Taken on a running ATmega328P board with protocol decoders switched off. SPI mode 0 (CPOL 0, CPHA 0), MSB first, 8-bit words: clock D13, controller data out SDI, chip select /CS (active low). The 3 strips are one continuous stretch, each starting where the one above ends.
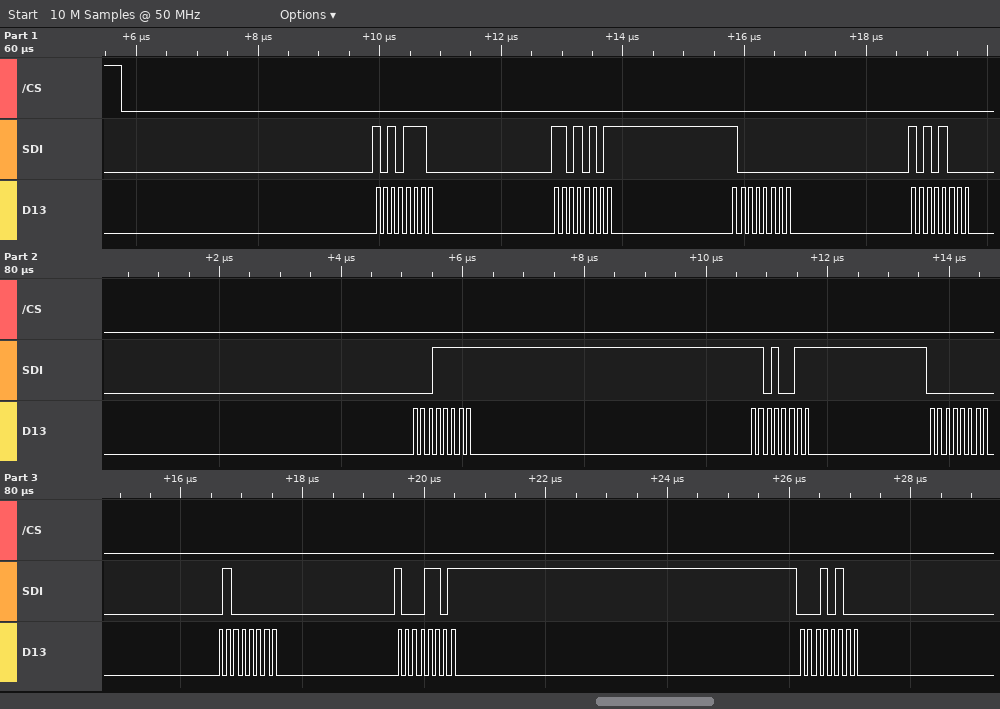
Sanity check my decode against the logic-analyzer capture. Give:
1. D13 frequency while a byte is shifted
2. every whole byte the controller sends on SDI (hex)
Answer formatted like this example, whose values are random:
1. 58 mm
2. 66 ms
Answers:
1. 8 MHz
2. AE D5 80 A8 1F D3 00 40 8D 14
